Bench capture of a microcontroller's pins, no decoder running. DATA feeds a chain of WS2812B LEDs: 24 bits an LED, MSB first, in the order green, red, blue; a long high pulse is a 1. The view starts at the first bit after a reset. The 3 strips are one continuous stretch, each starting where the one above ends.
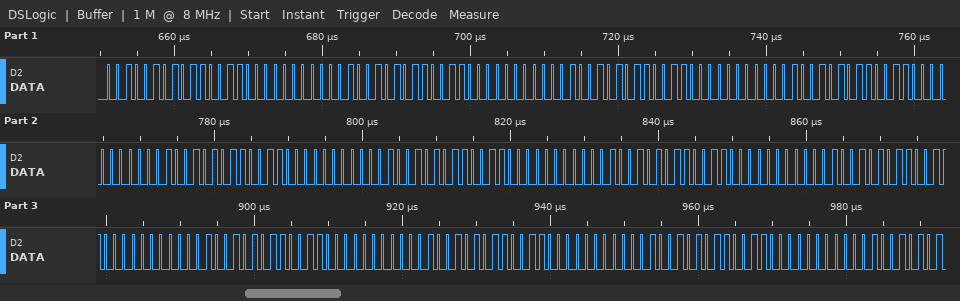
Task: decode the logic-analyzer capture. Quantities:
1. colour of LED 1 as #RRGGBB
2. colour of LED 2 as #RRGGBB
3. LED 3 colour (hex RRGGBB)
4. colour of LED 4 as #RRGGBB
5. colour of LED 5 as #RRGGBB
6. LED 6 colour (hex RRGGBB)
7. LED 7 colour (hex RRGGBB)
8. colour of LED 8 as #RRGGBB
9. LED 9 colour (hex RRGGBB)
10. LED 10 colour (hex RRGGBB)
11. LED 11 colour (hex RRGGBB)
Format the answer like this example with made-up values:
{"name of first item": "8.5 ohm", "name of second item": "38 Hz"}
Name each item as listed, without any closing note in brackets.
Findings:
{"colour of LED 1 as #RRGGBB": "#662500", "colour of LED 2 as #RRGGBB": "#662500", "LED 3 colour": "#662500", "colour of LED 4 as #RRGGBB": "#662500", "colour of LED 5 as #RRGGBB": "#662500", "LED 6 colour": "#662500", "LED 7 colour": "#662500", "colour of LED 8 as #RRGGBB": "#662500", "LED 9 colour": "#662500", "LED 10 colour": "#662500", "LED 11 colour": "#662500"}
